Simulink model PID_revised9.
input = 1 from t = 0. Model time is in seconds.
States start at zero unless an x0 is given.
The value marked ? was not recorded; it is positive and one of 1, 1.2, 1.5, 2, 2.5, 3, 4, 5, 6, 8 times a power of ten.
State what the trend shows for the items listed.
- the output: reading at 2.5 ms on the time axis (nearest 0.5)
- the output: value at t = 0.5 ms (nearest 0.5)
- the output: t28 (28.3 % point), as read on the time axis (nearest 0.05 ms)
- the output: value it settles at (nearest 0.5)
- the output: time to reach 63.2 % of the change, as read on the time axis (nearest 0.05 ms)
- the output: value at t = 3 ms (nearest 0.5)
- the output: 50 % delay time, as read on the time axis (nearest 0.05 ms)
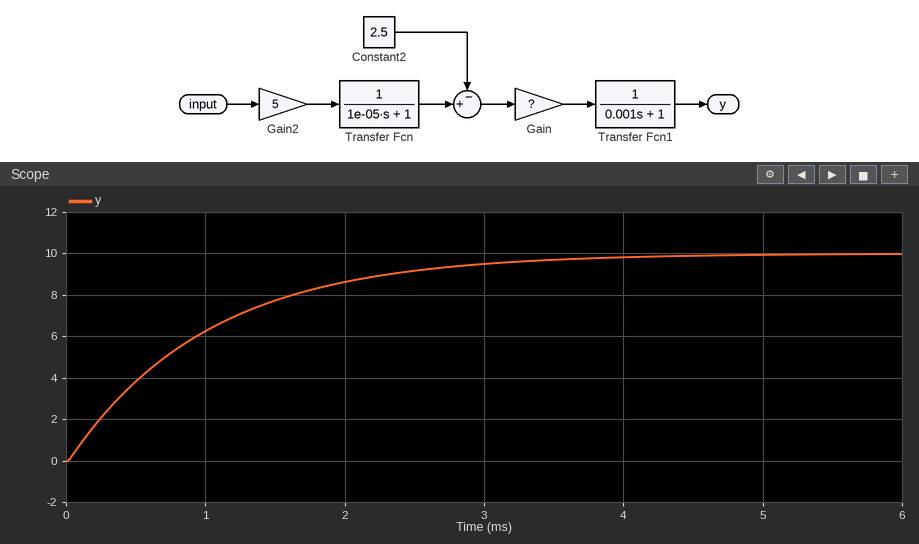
9.0
4.0
0.35 ms
10.0
1.00 ms
9.5
0.70 ms
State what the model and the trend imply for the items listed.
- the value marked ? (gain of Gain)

4
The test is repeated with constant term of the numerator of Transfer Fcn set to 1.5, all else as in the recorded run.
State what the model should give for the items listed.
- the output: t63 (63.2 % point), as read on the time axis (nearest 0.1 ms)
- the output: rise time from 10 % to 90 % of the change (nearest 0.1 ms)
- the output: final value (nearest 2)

1.0 ms
2.2 ms
20
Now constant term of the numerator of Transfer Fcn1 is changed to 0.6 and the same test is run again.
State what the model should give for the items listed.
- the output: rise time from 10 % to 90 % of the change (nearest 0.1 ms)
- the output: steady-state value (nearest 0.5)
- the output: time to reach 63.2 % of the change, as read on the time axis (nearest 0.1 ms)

2.2 ms
6.0
1.0 ms
